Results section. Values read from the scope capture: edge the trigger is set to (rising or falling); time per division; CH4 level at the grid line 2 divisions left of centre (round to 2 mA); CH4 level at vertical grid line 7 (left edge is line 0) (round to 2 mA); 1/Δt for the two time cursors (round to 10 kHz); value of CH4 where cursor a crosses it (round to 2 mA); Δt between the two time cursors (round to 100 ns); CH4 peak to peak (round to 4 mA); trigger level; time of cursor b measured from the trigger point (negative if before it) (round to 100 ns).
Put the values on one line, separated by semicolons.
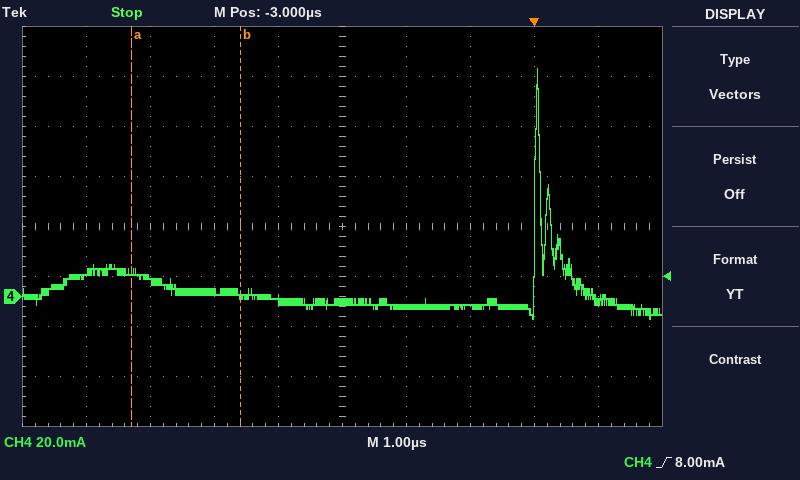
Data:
rising; 1 µs; 2 mA; -4 mA; 590 kHz; 10 mA; 1.7 µs; 100 mA; 8.00 mA; -4.6 µs
